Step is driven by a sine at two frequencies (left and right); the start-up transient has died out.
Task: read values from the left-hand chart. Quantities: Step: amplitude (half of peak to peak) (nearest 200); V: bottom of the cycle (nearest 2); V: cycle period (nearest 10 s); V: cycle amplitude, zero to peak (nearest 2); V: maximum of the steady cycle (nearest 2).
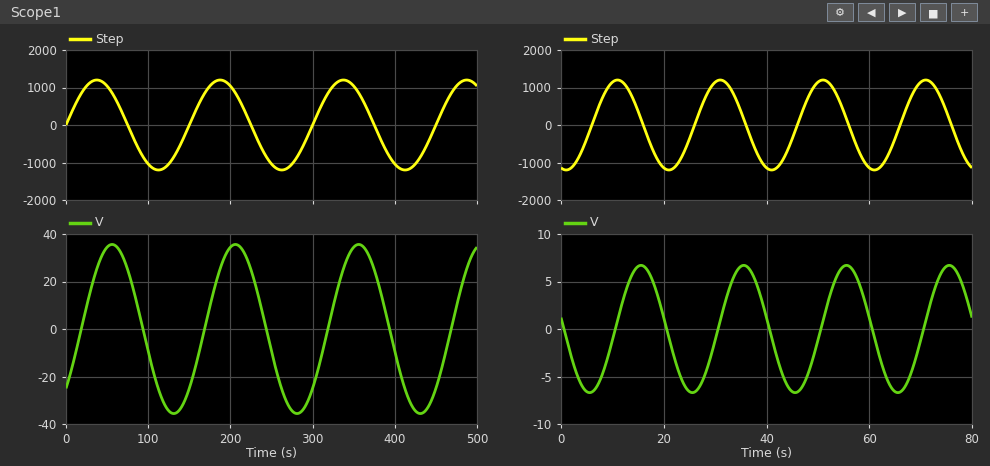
1200
-36
150 s
36
36
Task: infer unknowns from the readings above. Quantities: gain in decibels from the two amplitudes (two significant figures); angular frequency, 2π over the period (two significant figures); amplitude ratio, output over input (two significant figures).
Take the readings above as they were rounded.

-30 dB
0.042 rad/s
0.030
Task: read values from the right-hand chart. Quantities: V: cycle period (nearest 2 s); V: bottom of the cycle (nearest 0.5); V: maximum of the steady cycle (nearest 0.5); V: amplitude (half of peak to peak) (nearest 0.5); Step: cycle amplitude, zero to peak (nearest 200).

20 s
-6.5
6.5
6.5
1200
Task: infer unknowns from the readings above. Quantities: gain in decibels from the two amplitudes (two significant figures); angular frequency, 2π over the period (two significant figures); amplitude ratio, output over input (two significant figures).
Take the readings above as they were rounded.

-45 dB
0.31 rad/s
0.0054
